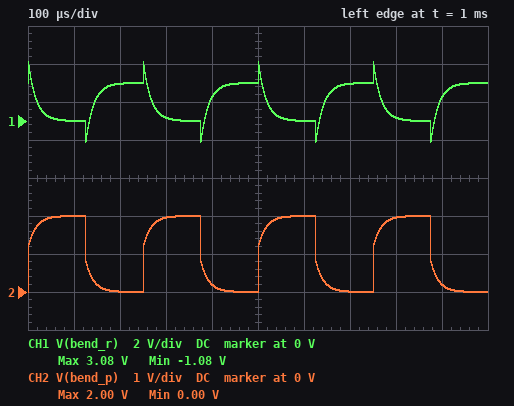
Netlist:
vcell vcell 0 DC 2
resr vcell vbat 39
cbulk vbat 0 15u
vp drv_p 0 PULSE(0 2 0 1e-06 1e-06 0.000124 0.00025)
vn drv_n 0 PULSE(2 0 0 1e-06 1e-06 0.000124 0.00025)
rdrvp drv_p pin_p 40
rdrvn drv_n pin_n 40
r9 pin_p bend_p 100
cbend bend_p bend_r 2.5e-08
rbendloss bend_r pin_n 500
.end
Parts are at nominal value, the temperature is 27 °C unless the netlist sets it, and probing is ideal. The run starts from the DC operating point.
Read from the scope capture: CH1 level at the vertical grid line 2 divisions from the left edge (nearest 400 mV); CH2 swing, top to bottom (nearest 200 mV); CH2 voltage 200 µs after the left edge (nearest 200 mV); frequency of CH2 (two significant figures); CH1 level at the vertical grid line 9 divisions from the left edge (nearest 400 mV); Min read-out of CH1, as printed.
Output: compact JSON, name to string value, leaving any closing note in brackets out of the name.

{"CH1 level at the vertical grid line 2 divisions from the left edge": "2.0 V", "CH2 swing, top to bottom": "2.0 V", "CH2 voltage 200 µs after the left edge": "0 V", "frequency of CH2": "4.0 kHz", "CH1 level at the vertical grid line 9 divisions from the left edge": "1.2 V", "Min read-out of CH1, as printed": "-1.08 V"}
